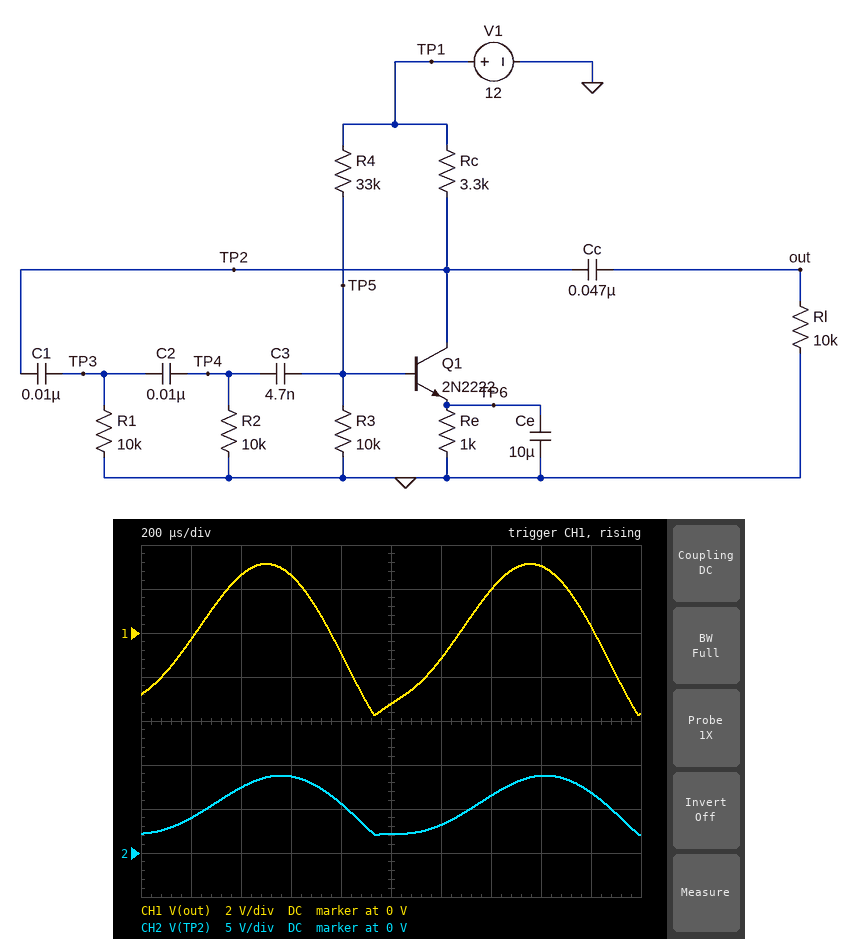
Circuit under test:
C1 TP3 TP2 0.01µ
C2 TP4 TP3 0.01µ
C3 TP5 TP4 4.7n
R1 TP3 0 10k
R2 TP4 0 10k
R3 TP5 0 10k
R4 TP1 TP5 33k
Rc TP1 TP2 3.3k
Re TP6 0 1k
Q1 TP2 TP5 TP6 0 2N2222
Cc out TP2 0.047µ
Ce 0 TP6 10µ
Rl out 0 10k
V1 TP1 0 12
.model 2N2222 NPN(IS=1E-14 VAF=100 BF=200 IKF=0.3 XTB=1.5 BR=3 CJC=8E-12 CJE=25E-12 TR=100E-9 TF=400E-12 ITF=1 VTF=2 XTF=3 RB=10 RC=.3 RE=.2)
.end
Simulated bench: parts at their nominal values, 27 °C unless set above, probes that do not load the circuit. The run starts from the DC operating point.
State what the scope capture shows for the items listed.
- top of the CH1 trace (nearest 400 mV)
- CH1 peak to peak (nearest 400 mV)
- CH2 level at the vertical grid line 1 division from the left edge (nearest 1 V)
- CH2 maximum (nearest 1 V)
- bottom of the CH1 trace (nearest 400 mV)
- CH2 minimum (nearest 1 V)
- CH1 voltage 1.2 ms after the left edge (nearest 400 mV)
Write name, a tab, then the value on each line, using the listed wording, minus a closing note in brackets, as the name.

top of the CH1 trace	3.2 V
CH1 peak to peak	6.8 V
CH2 level at the vertical grid line 1 division from the left edge	4 V
CH2 maximum	9 V
bottom of the CH1 trace	-3.6 V
CH2 minimum	2 V
CH1 voltage 1.2 ms after the left edge	-1.2 V
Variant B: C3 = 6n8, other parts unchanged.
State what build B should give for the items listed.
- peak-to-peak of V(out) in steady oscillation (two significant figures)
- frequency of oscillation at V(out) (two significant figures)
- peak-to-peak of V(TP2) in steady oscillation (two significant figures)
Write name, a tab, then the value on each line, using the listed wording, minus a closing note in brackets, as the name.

peak-to-peak of V(out) in steady oscillation	7.0 V
frequency of oscillation at V(out)	840 Hz
peak-to-peak of V(TP2) in steady oscillation	6.8 V
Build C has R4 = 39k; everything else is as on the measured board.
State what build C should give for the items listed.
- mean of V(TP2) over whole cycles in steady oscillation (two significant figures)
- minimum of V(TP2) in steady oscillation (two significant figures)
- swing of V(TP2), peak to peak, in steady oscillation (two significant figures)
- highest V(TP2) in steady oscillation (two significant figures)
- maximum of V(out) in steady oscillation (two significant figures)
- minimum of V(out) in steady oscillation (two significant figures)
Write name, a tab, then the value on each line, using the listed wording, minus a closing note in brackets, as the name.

mean of V(TP2) over whole cycles in steady oscillation	6.3 V
minimum of V(TP2) in steady oscillation	1.8 V
swing of V(TP2), peak to peak, in steady oscillation	8.6 V
highest V(TP2) in steady oscillation	10 V
maximum of V(out) in steady oscillation	4.2 V
minimum of V(out) in steady oscillation	-4.4 V
